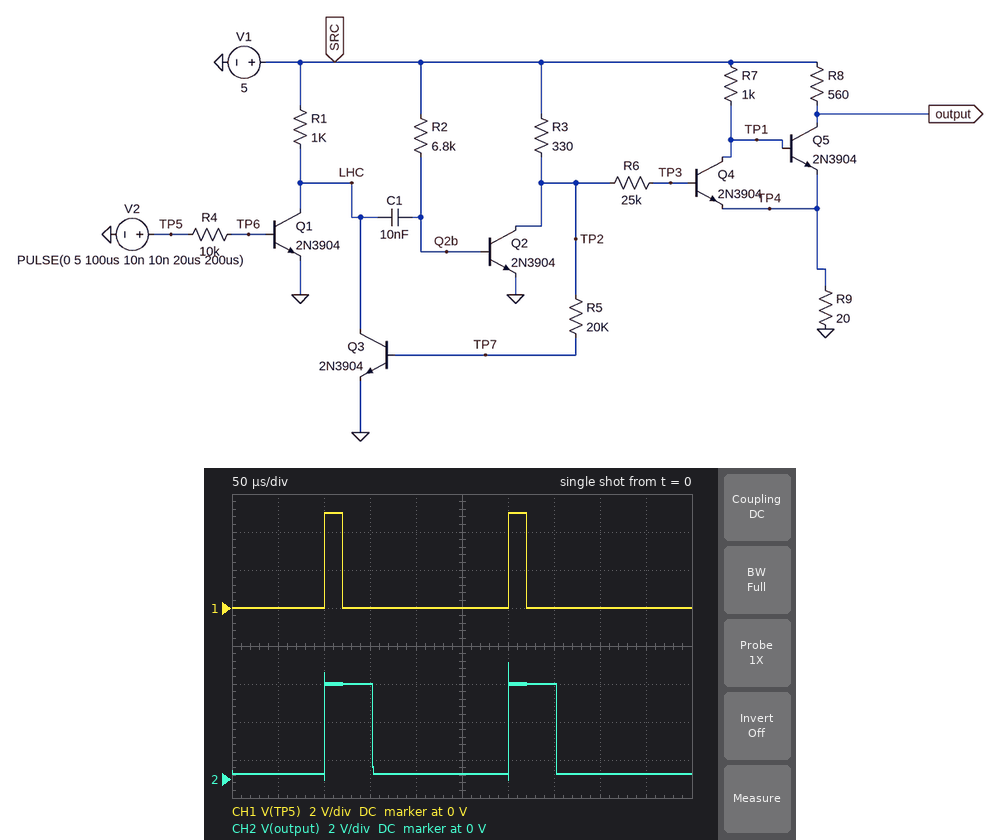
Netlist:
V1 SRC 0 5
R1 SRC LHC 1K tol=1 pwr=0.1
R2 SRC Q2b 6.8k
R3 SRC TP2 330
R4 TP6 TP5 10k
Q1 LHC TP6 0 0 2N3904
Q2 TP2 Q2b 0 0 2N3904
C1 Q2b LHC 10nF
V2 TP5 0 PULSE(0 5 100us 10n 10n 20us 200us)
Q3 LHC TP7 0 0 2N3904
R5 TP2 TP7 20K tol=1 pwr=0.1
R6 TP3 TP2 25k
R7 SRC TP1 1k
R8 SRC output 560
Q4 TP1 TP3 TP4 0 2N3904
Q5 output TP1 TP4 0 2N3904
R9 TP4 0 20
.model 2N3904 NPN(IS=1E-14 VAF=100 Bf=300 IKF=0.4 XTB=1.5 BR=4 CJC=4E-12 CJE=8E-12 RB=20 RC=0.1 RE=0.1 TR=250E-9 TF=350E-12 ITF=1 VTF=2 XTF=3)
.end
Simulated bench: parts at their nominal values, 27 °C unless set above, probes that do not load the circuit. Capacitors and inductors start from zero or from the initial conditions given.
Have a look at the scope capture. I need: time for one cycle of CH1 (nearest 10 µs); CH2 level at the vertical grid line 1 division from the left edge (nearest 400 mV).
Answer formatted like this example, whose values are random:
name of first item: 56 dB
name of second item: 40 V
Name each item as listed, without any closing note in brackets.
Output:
time for one cycle of CH1: 200 µs
CH2 level at the vertical grid line 1 division from the left edge: 400 mV
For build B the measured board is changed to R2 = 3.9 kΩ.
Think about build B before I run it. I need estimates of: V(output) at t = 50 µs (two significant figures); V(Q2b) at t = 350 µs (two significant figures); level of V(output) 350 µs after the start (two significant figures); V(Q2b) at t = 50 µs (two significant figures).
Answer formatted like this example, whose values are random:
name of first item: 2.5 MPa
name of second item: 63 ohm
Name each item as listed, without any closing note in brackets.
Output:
V(output) at t = 50 µs: 270 mV
V(Q2b) at t = 350 µs: 780 mV
level of V(output) 350 µs after the start: 270 mV
V(Q2b) at t = 50 µs: 760 mV
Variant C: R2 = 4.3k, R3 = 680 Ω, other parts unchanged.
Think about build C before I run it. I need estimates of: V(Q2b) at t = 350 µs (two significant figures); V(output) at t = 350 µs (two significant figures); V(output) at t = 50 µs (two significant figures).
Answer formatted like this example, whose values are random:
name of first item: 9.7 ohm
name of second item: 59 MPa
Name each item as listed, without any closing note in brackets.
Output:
V(Q2b) at t = 350 µs: 770 mV
V(output) at t = 350 µs: 270 mV
V(output) at t = 50 µs: 270 mV
